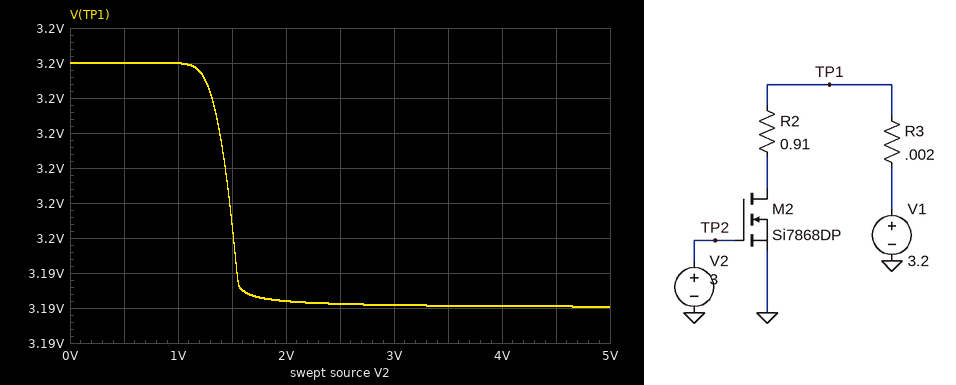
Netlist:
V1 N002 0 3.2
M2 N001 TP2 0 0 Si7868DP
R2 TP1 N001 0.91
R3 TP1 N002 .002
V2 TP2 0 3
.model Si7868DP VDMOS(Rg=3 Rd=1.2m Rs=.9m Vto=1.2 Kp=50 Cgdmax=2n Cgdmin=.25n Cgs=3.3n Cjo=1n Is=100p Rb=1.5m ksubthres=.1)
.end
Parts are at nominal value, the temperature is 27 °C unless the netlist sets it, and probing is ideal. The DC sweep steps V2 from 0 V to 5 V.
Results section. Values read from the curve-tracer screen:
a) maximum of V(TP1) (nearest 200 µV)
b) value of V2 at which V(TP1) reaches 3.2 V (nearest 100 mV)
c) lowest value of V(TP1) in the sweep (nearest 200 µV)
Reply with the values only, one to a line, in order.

3.2000 V
1.4 V
3.1930 V
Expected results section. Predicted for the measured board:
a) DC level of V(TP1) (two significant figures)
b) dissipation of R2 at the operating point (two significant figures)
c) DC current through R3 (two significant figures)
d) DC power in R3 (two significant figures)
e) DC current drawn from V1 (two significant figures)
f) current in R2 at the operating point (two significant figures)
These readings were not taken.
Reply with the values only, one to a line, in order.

3.2 V
11 W
3.5 A
24 mW
3.5 A
3.5 A
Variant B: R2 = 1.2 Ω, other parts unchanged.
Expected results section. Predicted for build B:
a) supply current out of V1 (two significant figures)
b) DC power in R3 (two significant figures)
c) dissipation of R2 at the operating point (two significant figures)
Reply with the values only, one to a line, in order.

2.6 A
14 mW
8.3 W
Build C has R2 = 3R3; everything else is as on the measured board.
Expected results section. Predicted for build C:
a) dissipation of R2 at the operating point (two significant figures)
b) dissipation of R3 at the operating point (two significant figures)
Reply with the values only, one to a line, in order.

3.1 W
1.9 mW
